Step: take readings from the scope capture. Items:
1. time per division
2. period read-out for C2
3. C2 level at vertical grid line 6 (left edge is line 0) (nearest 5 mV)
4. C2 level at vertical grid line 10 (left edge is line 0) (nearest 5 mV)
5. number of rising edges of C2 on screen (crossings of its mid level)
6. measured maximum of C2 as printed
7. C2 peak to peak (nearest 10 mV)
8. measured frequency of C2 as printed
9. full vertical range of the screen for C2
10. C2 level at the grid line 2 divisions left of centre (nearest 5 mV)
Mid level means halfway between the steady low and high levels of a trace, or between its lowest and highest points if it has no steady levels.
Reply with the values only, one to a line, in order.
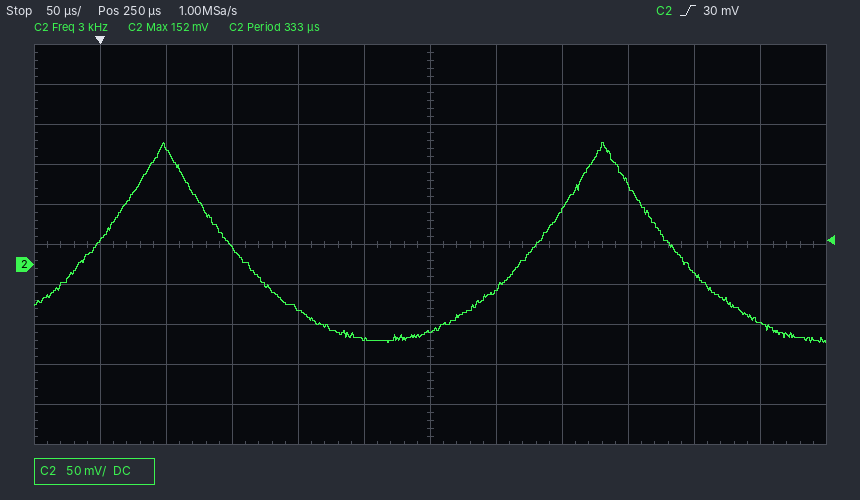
50 µs
333 µs
-85 mV
-10 mV
2
152 mV
250 mV
3 kHz
500 mV
-55 mV
